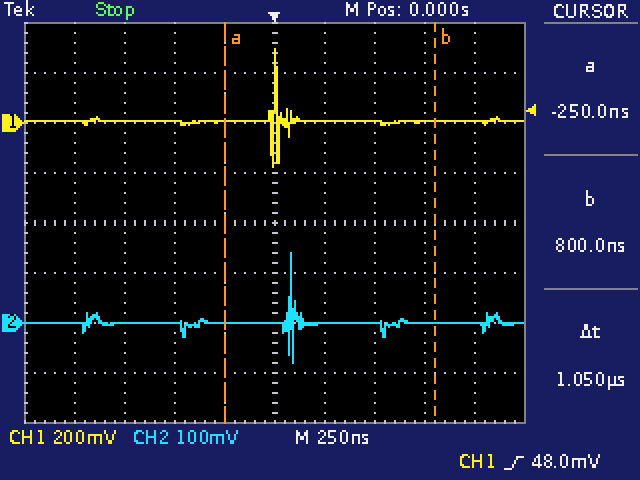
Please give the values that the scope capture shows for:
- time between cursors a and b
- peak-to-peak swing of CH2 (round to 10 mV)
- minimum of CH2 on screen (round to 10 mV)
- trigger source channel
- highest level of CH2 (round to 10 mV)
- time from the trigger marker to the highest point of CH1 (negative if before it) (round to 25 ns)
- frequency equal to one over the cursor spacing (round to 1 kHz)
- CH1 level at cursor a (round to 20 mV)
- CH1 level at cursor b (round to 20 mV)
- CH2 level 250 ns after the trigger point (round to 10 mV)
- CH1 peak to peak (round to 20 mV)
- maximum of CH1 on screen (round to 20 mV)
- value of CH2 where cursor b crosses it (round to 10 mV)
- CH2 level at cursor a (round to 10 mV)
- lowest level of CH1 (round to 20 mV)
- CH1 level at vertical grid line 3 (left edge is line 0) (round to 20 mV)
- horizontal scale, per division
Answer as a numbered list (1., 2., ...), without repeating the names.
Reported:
1. 1.05 µs
2. 220 mV
3. -80 mV
4. CH1
5. 140 mV
6. 0 ns
7. 952 kHz
8. 0 mV
9. 0 mV
10. 0 mV
11. 480 mV
12. 300 mV
13. 0 mV
14. 0 mV
15. -180 mV
16. 0 mV
17. 250 ns
